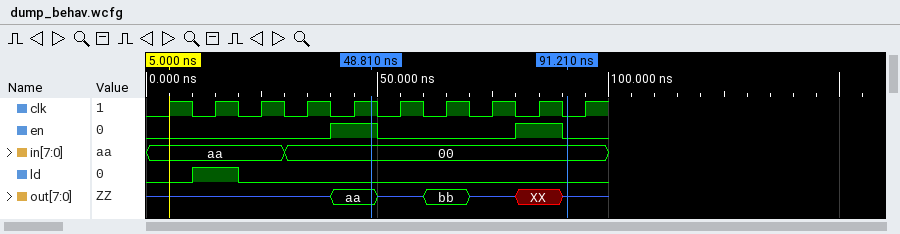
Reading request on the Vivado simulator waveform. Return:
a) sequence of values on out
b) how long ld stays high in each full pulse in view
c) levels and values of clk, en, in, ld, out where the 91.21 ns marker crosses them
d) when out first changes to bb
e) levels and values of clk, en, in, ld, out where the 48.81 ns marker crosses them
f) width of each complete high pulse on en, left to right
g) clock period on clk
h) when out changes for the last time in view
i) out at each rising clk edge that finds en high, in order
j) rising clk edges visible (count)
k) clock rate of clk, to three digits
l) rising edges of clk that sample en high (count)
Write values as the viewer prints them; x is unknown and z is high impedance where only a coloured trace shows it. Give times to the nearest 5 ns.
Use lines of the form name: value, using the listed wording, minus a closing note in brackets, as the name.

sequence of values on out: z, aa, z, bb, z, XX, z
how long ld stays high in each full pulse in view: 10 ns
levels and values of clk, en, in, ld, out where the 91.21 ns marker crosses them: clk=0, en=0, in=00, ld=0, out=z
when out first changes to bb: 60 ns
levels and values of clk, en, in, ld, out where the 48.81 ns marker crosses them: clk=1, en=1, in=00, ld=0, out=aa
width of each complete high pulse on en, left to right: 10 ns, 10 ns
clock period on clk: 10 ns
when out changes for the last time in view: 90 ns
out at each rising clk edge that finds en high, in order: aa, XX
rising clk edges visible: 10
clock rate of clk, to three digits: 100 MHz
rising edges of clk that sample en high: 2
